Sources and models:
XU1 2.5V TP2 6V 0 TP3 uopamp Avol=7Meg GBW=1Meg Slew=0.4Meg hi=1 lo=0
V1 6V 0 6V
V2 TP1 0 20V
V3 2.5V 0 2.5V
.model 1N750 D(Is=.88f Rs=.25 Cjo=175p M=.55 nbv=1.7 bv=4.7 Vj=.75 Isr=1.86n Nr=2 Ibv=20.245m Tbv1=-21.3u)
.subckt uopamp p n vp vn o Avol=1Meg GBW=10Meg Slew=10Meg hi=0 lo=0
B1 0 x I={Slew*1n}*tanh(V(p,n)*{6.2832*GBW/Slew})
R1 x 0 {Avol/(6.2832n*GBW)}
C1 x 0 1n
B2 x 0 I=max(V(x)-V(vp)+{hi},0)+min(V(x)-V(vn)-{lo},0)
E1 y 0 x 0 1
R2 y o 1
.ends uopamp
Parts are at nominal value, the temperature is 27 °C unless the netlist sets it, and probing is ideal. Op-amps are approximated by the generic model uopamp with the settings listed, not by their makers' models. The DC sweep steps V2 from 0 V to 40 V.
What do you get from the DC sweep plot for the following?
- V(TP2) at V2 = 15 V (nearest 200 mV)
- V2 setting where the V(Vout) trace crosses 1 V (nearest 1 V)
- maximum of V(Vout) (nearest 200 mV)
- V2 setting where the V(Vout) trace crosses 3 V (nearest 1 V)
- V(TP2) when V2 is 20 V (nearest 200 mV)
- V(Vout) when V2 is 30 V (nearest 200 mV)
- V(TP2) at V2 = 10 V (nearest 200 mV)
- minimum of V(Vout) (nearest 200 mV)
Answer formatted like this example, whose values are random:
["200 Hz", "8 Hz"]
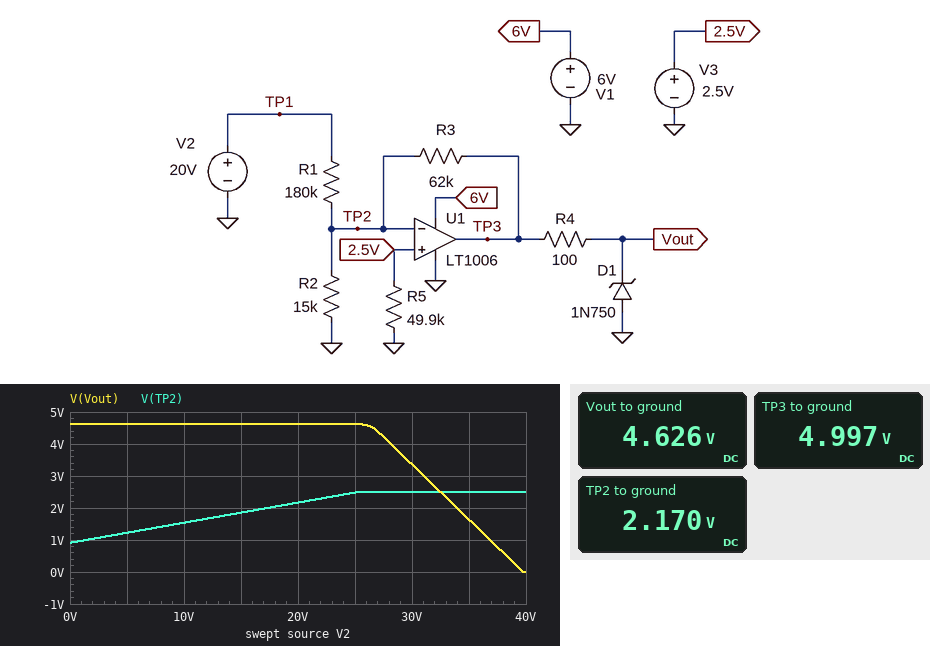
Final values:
["1.8 V", "37 V", "4.6 V", "31 V", "2.2 V", "3.4 V", "1.6 V", "0 V"]
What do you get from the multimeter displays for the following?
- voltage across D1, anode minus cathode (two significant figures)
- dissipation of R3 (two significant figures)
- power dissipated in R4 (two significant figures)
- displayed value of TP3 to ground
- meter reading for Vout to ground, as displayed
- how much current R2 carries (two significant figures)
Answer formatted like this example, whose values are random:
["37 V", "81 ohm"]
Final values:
["-4.6 V", "130 µW", "1.4 mW", "4.997 V", "4.626 V", "140 µA"]
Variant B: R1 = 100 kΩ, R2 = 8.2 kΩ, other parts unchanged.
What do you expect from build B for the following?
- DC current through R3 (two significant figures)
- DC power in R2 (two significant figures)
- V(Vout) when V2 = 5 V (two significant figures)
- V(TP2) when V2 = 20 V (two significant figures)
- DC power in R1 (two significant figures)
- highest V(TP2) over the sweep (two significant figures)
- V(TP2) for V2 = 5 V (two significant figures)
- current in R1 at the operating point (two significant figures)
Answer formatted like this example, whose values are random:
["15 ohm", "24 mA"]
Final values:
["50 µA", "440 µW", "4.6 V", "1.9 V", "3.3 mW", "2.7 V", "880 mV", "180 µA"]
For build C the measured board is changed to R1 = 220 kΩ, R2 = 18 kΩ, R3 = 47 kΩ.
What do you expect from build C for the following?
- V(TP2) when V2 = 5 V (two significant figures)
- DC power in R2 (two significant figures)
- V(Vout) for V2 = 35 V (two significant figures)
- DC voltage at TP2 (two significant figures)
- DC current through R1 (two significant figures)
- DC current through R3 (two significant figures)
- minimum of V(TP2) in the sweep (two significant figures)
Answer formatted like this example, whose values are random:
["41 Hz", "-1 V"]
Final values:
["1.6 V", "330 µW", "2.1 V", "2.4 V", "80 µA", "55 µA", "1.3 V"]
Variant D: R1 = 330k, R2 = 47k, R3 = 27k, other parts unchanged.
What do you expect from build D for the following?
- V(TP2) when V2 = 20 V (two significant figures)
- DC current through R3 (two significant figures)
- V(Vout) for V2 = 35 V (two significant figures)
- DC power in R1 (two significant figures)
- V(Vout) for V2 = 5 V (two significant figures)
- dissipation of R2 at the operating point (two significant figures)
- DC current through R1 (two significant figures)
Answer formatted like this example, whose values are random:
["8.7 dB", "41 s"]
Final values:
["2.5 V", "160 nA", "1.3 V", "930 µW", "3.7 V", "130 µW", "53 µA"]
